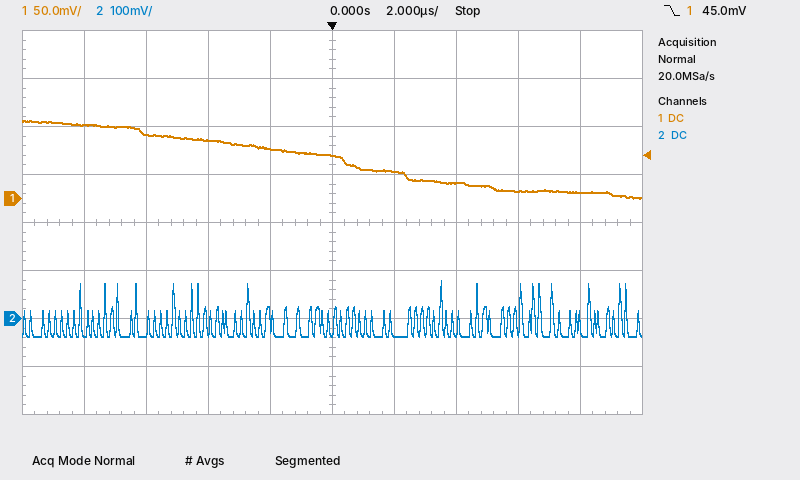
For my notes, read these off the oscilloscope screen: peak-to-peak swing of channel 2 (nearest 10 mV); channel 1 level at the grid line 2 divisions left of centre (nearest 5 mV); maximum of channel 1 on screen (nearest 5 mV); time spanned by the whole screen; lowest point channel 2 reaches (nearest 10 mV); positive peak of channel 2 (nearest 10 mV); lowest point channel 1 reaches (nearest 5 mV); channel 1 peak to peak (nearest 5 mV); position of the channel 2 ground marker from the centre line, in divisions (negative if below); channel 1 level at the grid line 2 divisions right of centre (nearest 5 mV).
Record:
120 mV
60 mV
80 mV
20 µs
-40 mV
80 mV
0 mV
80 mV
-2.0 div
15 mV
